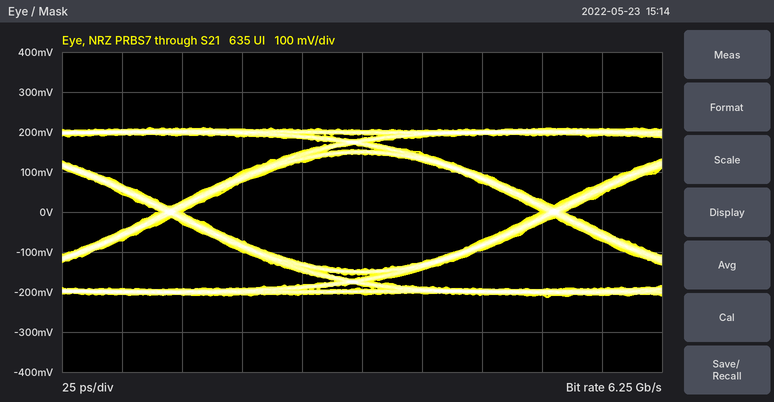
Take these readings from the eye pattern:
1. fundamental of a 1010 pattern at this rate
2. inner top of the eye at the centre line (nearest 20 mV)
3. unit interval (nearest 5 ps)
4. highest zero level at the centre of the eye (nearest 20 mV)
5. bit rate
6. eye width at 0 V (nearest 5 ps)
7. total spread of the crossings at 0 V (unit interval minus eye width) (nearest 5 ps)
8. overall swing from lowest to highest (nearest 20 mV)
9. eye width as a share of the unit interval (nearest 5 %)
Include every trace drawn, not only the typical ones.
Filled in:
3.125 GHz
140 mV
160 ps
-140 mV
6.25 Gb/s
150 ps
10 ps
420 mV
95 %
